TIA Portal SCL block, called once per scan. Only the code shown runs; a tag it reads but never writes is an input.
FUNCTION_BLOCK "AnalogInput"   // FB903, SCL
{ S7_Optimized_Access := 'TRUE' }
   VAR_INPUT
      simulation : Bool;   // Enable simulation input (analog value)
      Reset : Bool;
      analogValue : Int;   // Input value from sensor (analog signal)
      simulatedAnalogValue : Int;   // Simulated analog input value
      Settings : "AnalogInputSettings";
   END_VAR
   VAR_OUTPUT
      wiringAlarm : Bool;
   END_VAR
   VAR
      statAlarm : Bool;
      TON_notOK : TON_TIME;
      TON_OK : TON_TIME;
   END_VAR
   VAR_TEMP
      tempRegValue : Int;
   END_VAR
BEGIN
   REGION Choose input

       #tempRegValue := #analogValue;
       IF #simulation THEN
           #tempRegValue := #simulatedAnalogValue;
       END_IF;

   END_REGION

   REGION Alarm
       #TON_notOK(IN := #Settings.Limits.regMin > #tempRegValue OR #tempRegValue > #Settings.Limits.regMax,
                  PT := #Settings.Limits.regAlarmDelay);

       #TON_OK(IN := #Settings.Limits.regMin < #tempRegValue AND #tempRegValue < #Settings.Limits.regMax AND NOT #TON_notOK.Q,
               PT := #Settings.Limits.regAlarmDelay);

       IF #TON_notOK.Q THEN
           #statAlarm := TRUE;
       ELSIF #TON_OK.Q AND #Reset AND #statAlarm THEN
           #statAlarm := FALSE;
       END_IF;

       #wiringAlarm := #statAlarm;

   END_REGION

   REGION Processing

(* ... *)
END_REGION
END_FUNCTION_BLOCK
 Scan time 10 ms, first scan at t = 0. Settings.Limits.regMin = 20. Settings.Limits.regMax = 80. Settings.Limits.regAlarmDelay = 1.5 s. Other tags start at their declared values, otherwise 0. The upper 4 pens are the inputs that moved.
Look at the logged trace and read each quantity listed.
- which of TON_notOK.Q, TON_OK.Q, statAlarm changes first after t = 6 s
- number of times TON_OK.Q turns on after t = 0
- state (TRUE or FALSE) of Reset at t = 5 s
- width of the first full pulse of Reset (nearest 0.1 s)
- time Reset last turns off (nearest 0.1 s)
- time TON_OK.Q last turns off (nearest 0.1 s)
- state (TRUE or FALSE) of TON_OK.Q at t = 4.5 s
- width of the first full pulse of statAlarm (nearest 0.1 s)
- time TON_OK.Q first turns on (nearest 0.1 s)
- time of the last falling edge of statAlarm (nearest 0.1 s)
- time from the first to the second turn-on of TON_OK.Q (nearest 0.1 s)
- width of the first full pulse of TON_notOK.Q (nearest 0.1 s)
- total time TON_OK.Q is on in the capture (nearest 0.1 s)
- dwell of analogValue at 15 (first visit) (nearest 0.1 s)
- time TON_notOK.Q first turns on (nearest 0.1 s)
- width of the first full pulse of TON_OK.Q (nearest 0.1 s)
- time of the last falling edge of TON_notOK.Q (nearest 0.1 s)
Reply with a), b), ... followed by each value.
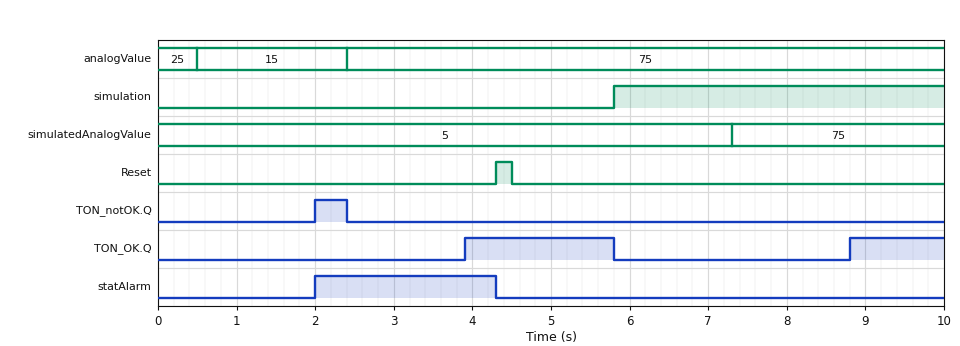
a) TON_OK.Q
b) 2
c) FALSE
d) 0.2 s
e) 4.5 s
f) 5.8 s
g) TRUE
h) 2.3 s
i) 3.9 s
j) 4.3 s
k) 4.9 s
l) 0.4 s
m) 3.1 s
n) 1.9 s
o) 2.0 s
p) 1.9 s
q) 2.4 s
